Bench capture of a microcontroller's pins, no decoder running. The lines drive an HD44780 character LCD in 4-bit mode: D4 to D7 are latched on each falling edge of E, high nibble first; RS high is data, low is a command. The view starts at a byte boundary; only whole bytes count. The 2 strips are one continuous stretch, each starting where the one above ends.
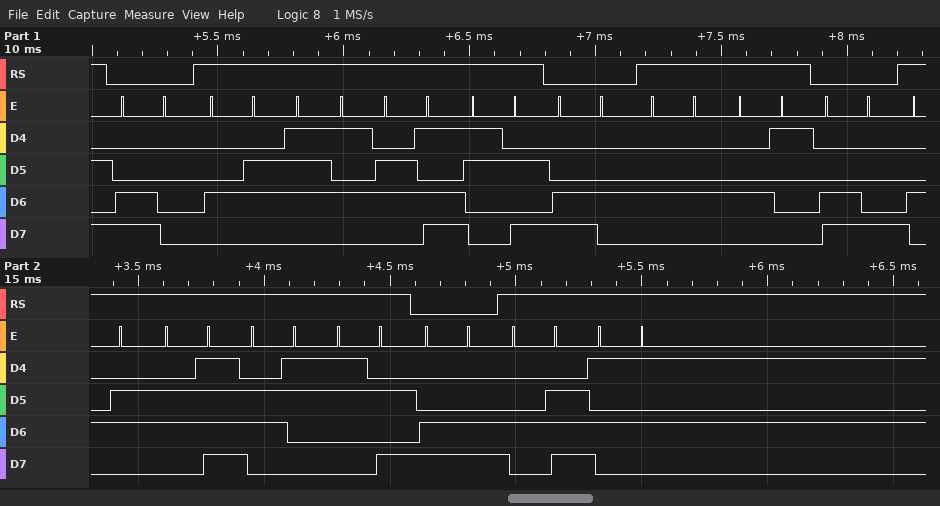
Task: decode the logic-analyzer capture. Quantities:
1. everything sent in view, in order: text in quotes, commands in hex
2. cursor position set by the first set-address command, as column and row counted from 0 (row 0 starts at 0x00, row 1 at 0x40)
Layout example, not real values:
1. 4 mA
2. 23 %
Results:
1. 0xC0 "Fum:" 0xC4 "DA" 0xC8 "Foc:" 0xCC "NU"
2. column 0, row 1
